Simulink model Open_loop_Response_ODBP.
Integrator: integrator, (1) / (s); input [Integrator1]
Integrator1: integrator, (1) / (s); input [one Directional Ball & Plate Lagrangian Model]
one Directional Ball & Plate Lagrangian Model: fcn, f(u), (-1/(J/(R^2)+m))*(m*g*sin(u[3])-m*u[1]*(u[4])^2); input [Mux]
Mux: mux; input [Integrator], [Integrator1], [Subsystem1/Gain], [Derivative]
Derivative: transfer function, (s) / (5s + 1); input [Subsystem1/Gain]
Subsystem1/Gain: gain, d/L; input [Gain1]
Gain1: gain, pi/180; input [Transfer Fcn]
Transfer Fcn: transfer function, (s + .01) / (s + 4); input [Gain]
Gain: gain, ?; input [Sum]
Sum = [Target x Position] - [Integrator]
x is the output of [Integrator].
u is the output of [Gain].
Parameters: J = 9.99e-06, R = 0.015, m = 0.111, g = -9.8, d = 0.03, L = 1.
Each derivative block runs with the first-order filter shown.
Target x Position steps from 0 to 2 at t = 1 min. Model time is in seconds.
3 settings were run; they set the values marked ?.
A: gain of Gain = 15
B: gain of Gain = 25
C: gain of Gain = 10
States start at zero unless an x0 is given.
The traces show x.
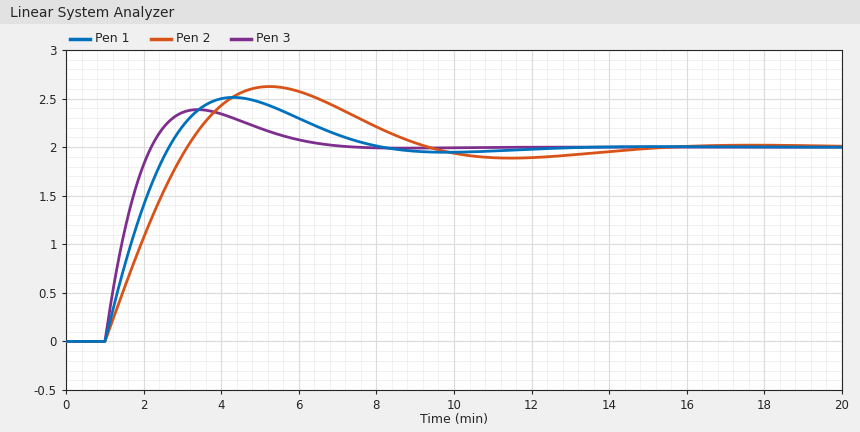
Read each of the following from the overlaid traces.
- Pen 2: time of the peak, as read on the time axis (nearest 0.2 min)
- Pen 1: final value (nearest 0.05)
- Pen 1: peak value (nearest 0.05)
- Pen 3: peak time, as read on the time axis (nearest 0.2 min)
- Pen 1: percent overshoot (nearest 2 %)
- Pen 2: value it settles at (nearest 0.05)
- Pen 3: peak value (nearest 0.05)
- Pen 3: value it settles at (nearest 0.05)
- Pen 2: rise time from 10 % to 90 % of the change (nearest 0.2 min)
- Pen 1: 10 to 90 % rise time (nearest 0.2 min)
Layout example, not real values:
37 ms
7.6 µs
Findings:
5.2 min
2.00
2.50
3.4 min
26 %
2.00
2.40
2.00
1.6 min
1.2 min
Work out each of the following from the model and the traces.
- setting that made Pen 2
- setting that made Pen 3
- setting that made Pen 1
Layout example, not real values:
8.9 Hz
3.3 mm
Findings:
C
B
A
